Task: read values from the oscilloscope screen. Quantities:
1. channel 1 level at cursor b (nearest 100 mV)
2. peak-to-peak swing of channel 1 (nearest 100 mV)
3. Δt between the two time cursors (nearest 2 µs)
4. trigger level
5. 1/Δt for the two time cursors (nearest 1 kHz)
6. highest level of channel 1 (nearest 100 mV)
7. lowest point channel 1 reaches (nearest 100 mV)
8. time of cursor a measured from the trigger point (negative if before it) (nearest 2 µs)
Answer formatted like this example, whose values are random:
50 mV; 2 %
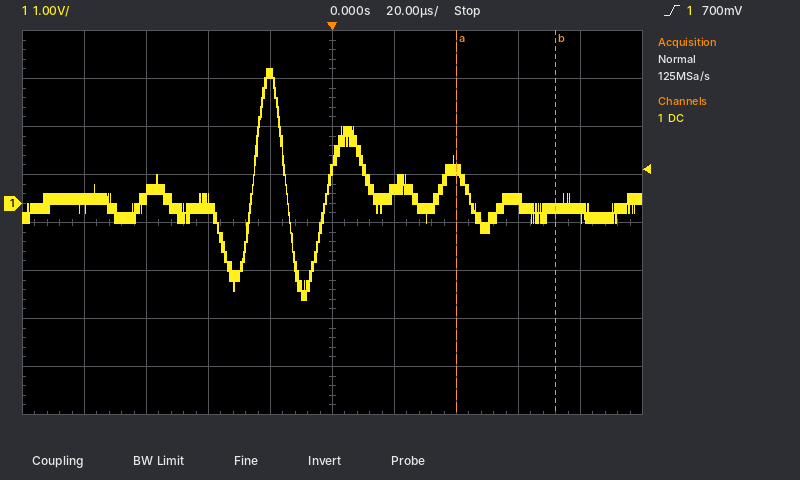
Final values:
-100 mV; 4.8 V; 32 µs; 700 mV; 31 kHz; 2.8 V; -2.0 V; +40 µs
